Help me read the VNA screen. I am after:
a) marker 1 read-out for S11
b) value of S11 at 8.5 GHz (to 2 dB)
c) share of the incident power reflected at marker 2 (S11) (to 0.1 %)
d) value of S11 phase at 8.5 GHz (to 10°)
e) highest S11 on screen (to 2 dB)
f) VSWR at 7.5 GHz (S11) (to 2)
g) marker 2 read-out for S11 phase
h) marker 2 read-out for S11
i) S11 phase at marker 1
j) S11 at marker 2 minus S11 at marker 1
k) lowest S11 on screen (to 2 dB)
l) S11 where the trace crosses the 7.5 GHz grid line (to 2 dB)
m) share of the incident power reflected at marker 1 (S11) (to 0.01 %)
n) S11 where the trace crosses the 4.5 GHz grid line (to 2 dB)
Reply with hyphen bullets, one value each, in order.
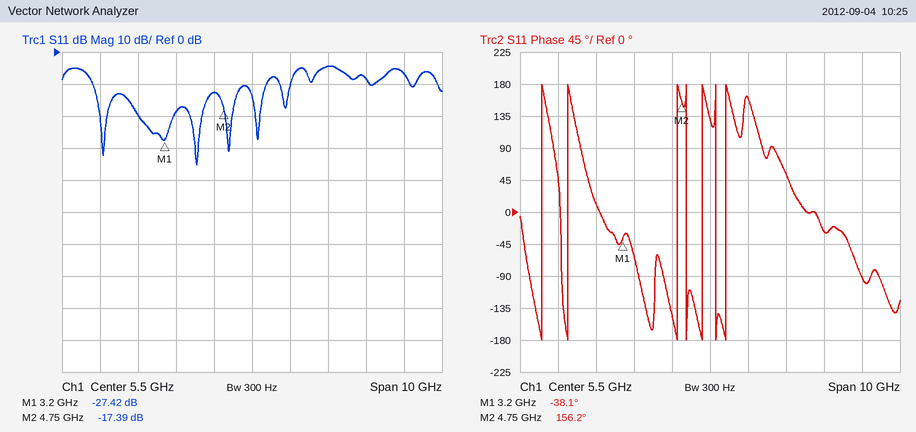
- -27.42 dB
- -8 dB
- 1.8 %
- -30°
- -4 dB
- 4
- 156.2°
- -17.39 dB
- -38.1°
- 10.03 dB
- -36 dB
- -4 dB
- 0.18 %
- -12 dB
